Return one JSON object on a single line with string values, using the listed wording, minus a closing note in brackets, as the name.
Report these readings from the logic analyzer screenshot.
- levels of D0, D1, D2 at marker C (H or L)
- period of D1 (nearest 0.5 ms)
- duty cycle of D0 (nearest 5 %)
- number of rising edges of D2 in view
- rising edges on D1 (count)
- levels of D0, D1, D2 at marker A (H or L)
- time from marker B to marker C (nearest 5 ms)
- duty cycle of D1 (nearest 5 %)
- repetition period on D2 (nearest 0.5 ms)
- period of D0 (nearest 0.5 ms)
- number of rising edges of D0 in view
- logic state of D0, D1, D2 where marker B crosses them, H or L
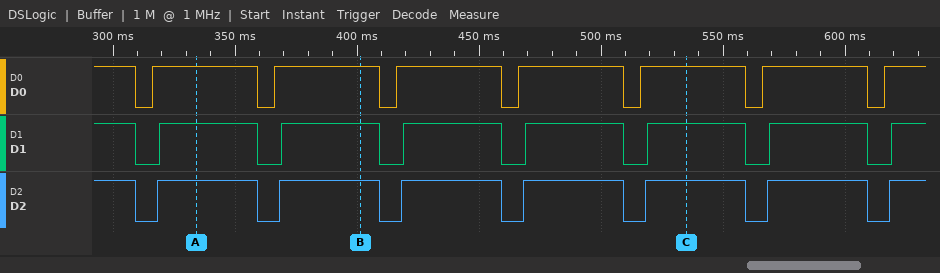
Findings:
{"levels of D0, D1, D2 at marker C": "D0=H, D1=H, D2=H", "period of D1": "50 ms", "duty cycle of D0": "85 %", "number of rising edges of D2 in view": "7", "rising edges on D1": "7", "levels of D0, D1, D2 at marker A": "D0=H, D1=H, D2=H", "time from marker B to marker C": "135 ms", "duty cycle of D1": "80 %", "repetition period on D2": "50 ms", "period of D0": "50 ms", "number of rising edges of D0 in view": "7", "logic state of D0, D1, D2 where marker B crosses them, H or L": "D0=H, D1=H, D2=H"}
